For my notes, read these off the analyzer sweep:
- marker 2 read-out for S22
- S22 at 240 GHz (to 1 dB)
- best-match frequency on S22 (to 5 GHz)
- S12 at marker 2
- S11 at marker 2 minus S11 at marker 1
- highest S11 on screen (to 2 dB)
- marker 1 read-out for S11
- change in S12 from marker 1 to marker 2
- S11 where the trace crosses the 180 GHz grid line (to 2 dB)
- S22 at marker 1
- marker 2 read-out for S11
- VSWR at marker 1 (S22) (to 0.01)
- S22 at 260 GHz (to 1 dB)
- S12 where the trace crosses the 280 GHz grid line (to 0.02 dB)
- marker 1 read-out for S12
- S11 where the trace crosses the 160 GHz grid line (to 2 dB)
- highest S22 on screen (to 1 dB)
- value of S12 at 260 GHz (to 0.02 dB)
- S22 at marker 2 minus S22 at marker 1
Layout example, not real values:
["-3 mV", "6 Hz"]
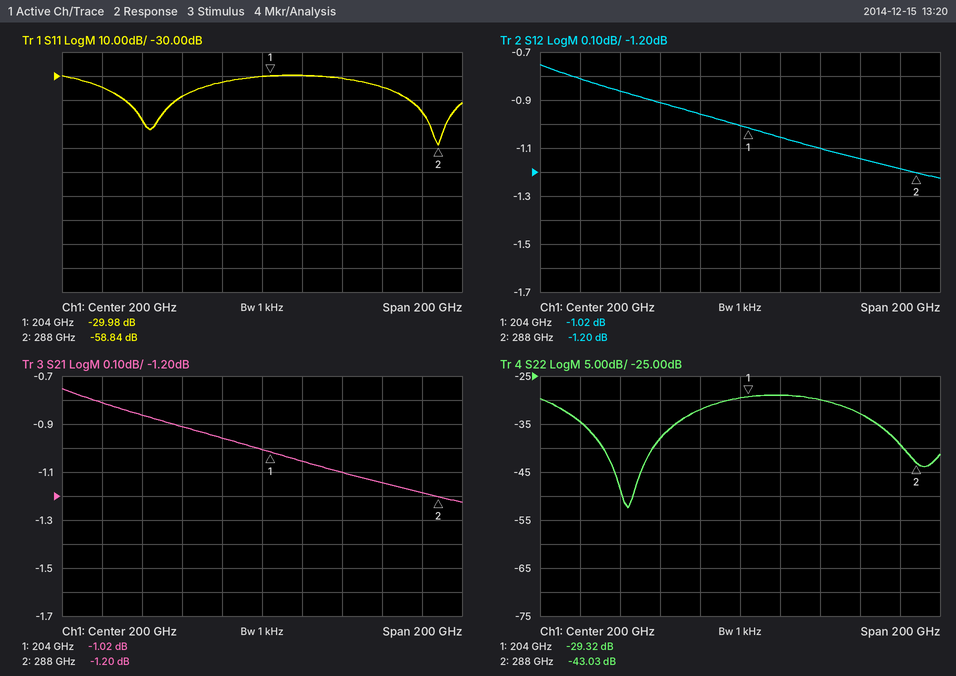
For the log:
["-43.03 dB", "-30 dB", "145 GHz", "-1.20 dB", "-28.86 dB", "-30 dB", "-29.98 dB", "-0.18 dB", "-32 dB", "-29.32 dB", "-58.84 dB", "1.07", "-33 dB", "-1.18 dB", "-1.02 dB", "-38 dB", "-29 dB", "-1.14 dB", "-13.71 dB"]
